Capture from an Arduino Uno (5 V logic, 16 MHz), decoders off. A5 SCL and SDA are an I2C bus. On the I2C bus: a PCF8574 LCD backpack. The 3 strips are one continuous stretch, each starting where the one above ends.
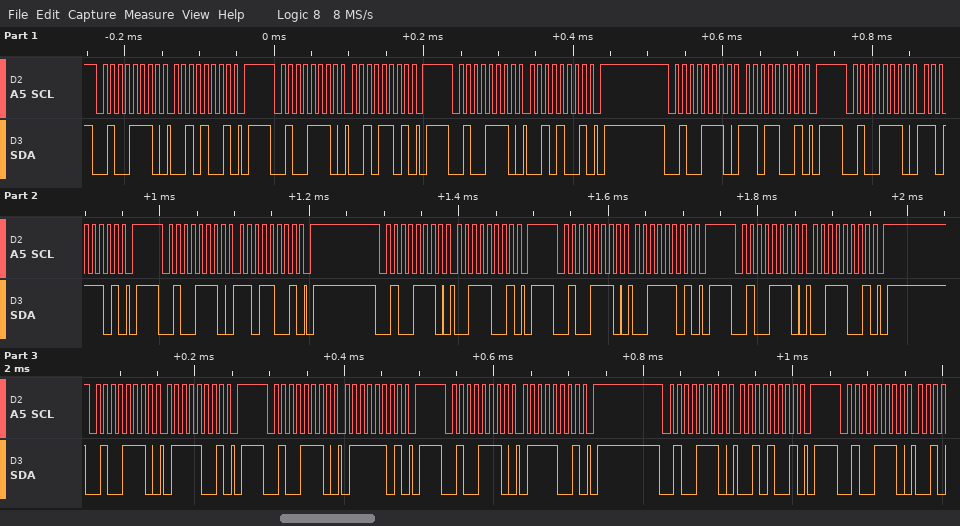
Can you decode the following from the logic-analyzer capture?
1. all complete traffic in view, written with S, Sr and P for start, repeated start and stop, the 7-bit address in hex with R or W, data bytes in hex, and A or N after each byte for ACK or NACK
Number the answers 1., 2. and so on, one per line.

1. S 27W A 29 A P S 27W A 2D A P S 27W A 29 A P S 27W A D9 A P S 27W A DD A P S 27W A D9 A P S 27W A 39 A P S 27W A 3D A P S 27W A 39 A P S 27W A 79 A P S 27W A 7D A P S 27W A 79 A P S 27W A 29 A P S 27W A
